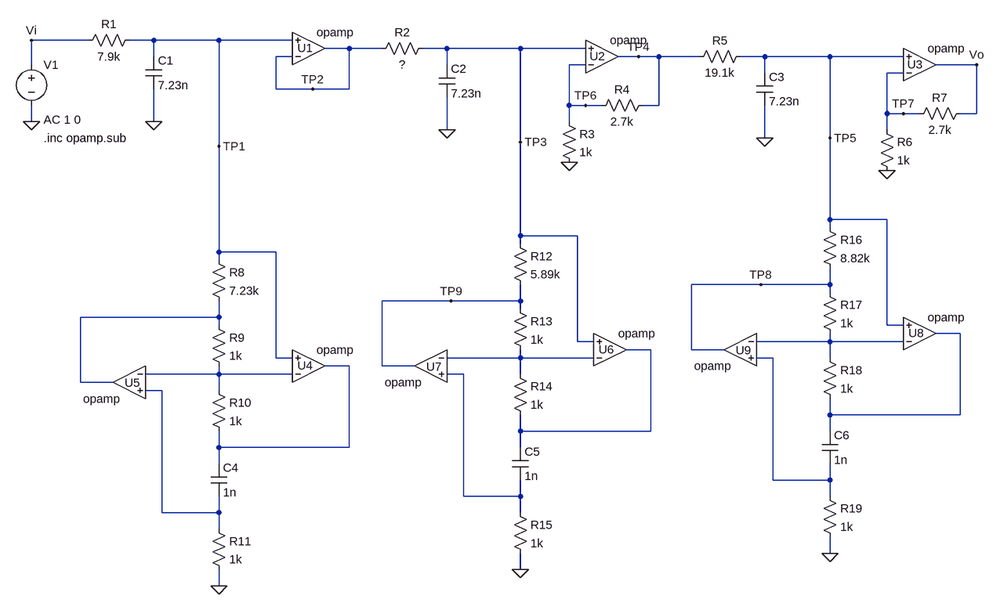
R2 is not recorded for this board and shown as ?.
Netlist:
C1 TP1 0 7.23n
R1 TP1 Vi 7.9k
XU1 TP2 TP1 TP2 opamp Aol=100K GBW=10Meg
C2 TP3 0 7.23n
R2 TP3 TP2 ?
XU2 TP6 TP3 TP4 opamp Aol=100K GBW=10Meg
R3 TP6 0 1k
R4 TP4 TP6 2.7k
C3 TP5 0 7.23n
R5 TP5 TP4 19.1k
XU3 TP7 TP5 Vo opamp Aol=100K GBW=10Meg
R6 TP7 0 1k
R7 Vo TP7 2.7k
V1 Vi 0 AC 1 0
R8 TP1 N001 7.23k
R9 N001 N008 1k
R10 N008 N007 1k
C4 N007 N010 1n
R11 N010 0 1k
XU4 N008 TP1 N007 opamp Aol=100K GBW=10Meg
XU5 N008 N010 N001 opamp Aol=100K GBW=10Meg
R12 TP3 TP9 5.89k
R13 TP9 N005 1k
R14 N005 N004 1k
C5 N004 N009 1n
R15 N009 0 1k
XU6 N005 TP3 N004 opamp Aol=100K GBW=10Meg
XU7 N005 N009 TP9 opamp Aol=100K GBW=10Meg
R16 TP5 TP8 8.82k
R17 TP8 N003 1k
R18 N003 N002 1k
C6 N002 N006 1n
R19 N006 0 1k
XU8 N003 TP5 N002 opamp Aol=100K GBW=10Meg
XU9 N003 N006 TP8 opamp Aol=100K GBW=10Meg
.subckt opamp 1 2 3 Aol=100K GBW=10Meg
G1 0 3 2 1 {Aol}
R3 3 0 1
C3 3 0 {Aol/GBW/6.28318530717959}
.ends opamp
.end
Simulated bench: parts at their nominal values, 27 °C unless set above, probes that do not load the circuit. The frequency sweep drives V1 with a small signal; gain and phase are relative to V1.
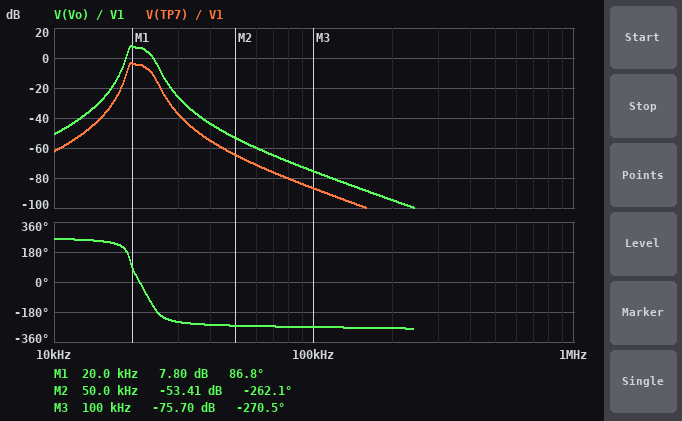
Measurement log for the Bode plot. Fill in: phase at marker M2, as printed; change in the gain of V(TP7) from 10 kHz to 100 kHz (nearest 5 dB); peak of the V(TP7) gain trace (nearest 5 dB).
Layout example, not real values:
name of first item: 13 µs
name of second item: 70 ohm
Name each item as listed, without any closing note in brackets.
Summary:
phase at marker M2, as printed: -262.1 deg
change in the gain of V(TP7) from 10 kHz to 100 kHz: -25 dB
peak of the V(TP7) gain trace: -5 dB
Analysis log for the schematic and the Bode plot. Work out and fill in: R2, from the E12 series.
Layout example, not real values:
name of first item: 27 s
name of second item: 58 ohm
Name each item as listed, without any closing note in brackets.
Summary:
R2, from the E12 series: 6.8 kΩ
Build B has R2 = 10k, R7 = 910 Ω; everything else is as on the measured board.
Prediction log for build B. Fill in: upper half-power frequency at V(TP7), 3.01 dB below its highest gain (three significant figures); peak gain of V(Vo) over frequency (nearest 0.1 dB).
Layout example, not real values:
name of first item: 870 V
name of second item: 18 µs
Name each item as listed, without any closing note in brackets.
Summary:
upper half-power frequency at V(TP7), 3.01 dB below its highest gain: 23.5 kHz
peak gain of V(Vo) over frequency: -0.9 dB
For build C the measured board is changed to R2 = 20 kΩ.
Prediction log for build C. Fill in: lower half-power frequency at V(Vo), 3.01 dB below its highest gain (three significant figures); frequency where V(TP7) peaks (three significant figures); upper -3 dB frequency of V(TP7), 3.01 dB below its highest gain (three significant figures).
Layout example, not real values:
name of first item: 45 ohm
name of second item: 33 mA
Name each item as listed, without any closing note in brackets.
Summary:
lower half-power frequency at V(Vo), 3.01 dB below its highest gain: 19.5 kHz
frequency where V(TP7) peaks: 23.8 kHz
upper -3 dB frequency of V(TP7), 3.01 dB below its highest gain: 24.3 kHz
